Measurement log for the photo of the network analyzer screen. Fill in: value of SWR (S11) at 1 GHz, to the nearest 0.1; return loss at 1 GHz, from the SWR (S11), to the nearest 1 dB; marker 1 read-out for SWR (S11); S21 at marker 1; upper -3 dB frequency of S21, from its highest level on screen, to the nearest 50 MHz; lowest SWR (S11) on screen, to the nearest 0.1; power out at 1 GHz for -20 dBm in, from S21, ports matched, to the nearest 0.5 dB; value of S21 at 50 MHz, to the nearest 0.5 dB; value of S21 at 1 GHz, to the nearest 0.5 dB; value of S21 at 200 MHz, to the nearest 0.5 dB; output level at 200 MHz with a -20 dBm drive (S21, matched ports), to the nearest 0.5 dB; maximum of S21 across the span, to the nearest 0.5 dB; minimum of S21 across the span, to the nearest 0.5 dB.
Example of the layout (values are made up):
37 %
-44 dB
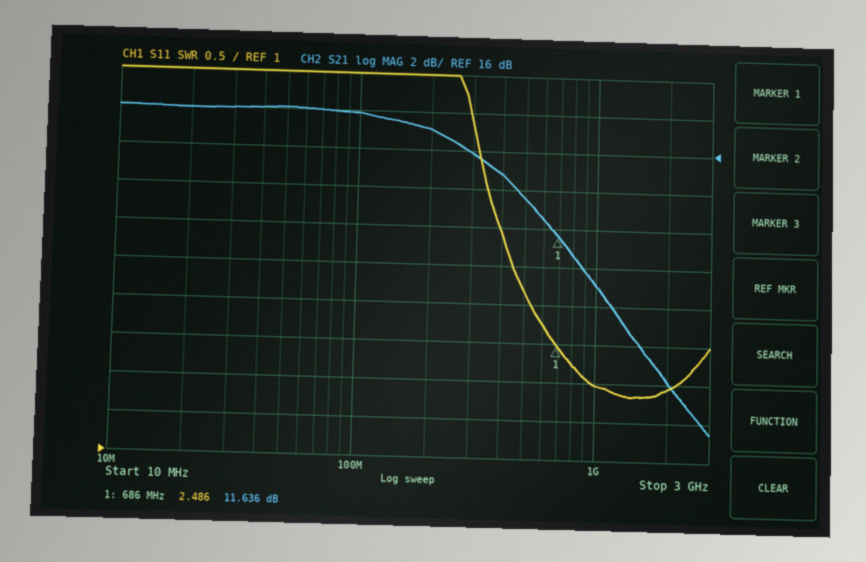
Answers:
2.0
10 dB
2.486
11.636 dB
350 MHz
1.8
-11.0 dBm
18.0 dB
9.0 dB
17.0 dB
-3.0 dBm
18.0 dB
1.5 dB
